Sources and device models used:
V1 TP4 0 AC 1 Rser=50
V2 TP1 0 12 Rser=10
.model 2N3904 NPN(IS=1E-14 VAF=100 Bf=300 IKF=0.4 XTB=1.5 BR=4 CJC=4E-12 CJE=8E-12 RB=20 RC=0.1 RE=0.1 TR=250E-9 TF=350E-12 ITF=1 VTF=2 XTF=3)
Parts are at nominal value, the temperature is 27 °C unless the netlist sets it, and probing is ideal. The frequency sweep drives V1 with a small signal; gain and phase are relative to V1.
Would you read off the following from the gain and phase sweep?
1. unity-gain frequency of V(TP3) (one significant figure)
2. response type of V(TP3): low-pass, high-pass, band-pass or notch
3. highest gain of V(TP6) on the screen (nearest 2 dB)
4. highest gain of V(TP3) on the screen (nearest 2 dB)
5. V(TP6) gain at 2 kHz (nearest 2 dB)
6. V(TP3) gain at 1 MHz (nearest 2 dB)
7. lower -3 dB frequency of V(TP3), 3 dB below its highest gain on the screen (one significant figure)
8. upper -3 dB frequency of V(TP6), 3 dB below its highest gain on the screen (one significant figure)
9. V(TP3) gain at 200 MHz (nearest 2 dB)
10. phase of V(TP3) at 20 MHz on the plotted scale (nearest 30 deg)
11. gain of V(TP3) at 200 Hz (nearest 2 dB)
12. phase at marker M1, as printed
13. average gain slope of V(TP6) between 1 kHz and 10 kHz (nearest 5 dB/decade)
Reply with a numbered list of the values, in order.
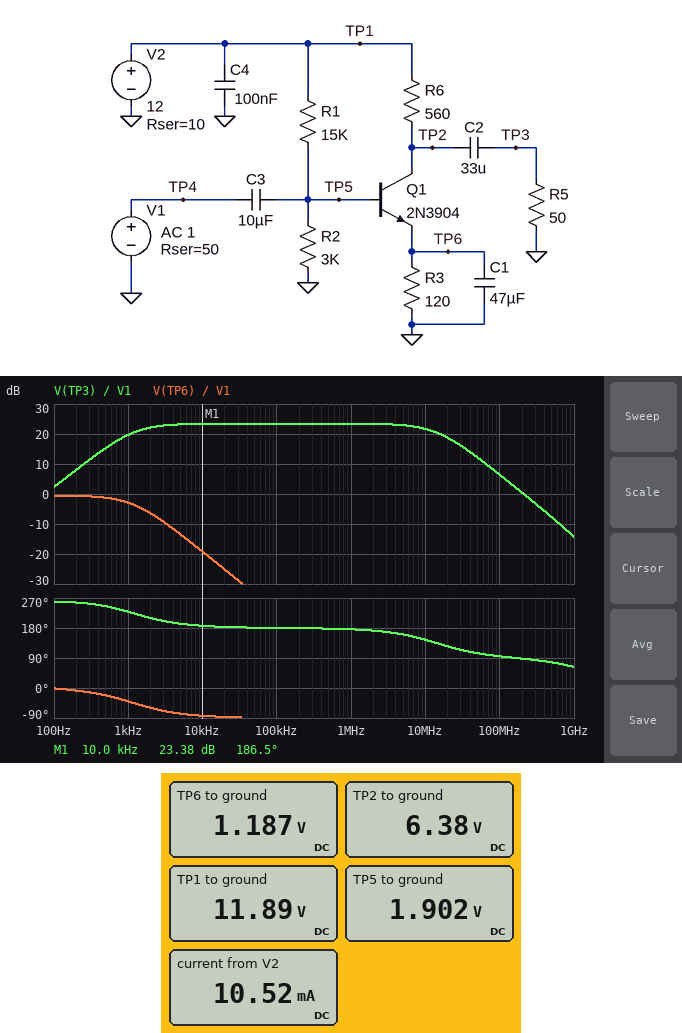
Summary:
1. 200 MHz
2. band-pass
3. 0 dB
4. 24 dB
5. -6 dB
6. 24 dB
7. 1 kHz
8. 1 kHz
9. 0 dB
10. 120 deg
11. 8 dB
12. 186.5 deg
13. -15 dB/decade
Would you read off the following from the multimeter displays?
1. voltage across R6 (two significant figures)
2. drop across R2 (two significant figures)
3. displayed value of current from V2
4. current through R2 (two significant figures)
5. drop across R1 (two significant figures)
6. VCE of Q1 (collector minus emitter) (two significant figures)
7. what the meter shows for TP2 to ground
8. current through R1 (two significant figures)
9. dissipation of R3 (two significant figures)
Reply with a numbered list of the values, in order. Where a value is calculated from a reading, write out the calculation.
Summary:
1. 11.89 V - 6.38 V = 5.5 V
2. 1.902 V = 1.9 V
3. 10.52 mA
4. (1.902 V) / 3 kΩ = 630 µA
5. 11.89 V - 1.902 V = 10 V
6. 6.38 V - 1.187 V = 5.2 V
7. 6.38 V
8. (11.89 V - 1.902 V) / 15 kΩ = 670 µA
9. (1.187 V)^2 / 120 Ω = 12 mW
